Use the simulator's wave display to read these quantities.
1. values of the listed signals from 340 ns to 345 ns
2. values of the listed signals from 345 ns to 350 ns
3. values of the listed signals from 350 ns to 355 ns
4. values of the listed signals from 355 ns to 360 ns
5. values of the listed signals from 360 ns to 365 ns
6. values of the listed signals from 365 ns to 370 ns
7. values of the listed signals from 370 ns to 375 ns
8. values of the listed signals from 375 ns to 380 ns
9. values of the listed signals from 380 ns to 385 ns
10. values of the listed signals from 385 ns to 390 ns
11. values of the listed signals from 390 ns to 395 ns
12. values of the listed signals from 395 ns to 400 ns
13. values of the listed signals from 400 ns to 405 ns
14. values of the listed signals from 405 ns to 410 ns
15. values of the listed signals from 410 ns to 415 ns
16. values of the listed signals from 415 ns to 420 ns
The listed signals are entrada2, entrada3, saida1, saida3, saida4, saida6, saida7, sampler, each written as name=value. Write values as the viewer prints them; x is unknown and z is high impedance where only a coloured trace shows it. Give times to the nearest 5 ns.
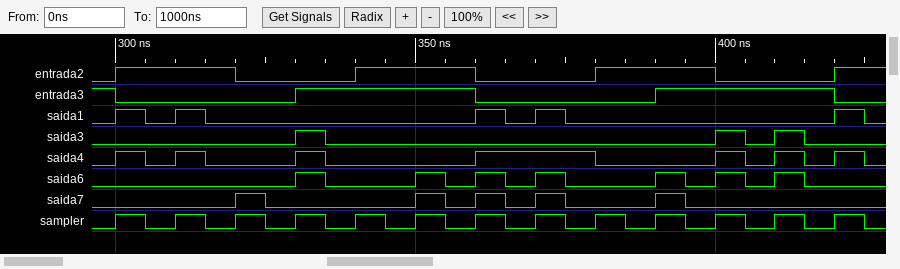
entrada2=1, entrada3=1, saida1=0, saida3=0, saida4=0, saida6=0, saida7=0, sampler=1
entrada2=1, entrada3=1, saida1=0, saida3=0, saida4=0, saida6=0, saida7=0, sampler=0
entrada2=1, entrada3=1, saida1=0, saida3=0, saida4=0, saida6=1, saida7=1, sampler=1
entrada2=1, entrada3=1, saida1=0, saida3=0, saida4=0, saida6=0, saida7=0, sampler=0
entrada2=0, entrada3=0, saida1=1, saida3=0, saida4=1, saida6=1, saida7=1, sampler=1
entrada2=0, entrada3=0, saida1=0, saida3=0, saida4=1, saida6=0, saida7=0, sampler=0
entrada2=0, entrada3=0, saida1=1, saida3=0, saida4=1, saida6=1, saida7=1, sampler=1
entrada2=0, entrada3=0, saida1=0, saida3=0, saida4=1, saida6=0, saida7=0, sampler=0
entrada2=1, entrada3=0, saida1=0, saida3=0, saida4=0, saida6=0, saida7=0, sampler=1
entrada2=1, entrada3=0, saida1=0, saida3=0, saida4=0, saida6=0, saida7=0, sampler=0
entrada2=1, entrada3=1, saida1=0, saida3=0, saida4=0, saida6=1, saida7=1, sampler=1
entrada2=1, entrada3=1, saida1=0, saida3=0, saida4=0, saida6=0, saida7=0, sampler=0
entrada2=0, entrada3=1, saida1=0, saida3=1, saida4=1, saida6=1, saida7=0, sampler=1
entrada2=0, entrada3=1, saida1=0, saida3=0, saida4=0, saida6=0, saida7=0, sampler=0
entrada2=0, entrada3=1, saida1=0, saida3=1, saida4=1, saida6=1, saida7=0, sampler=1
entrada2=0, entrada3=1, saida1=0, saida3=0, saida4=0, saida6=0, saida7=0, sampler=0
